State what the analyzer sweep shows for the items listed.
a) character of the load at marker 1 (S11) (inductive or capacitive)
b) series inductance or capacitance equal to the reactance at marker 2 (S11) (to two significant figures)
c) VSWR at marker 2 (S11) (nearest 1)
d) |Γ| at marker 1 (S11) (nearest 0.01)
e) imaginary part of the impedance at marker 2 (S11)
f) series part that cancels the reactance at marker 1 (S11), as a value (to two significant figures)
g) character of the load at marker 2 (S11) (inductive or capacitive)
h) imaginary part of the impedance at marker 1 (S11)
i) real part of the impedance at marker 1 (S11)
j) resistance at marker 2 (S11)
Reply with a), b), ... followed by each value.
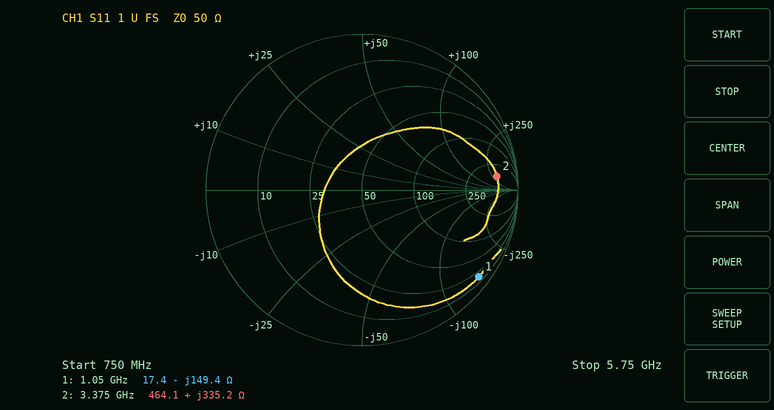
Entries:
a) capacitive
b) 16 nH
c) 14
d) 0.93
e) +335.2 Ω
f) 23 nH
g) inductive
h) -149.4 Ω
i) 17.4 Ω
j) 464.1 Ω
